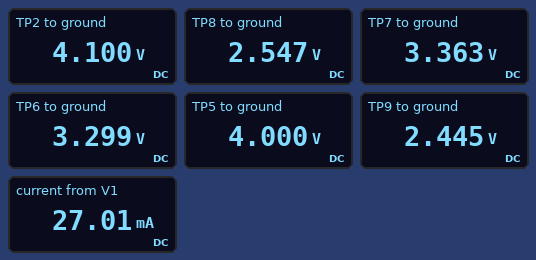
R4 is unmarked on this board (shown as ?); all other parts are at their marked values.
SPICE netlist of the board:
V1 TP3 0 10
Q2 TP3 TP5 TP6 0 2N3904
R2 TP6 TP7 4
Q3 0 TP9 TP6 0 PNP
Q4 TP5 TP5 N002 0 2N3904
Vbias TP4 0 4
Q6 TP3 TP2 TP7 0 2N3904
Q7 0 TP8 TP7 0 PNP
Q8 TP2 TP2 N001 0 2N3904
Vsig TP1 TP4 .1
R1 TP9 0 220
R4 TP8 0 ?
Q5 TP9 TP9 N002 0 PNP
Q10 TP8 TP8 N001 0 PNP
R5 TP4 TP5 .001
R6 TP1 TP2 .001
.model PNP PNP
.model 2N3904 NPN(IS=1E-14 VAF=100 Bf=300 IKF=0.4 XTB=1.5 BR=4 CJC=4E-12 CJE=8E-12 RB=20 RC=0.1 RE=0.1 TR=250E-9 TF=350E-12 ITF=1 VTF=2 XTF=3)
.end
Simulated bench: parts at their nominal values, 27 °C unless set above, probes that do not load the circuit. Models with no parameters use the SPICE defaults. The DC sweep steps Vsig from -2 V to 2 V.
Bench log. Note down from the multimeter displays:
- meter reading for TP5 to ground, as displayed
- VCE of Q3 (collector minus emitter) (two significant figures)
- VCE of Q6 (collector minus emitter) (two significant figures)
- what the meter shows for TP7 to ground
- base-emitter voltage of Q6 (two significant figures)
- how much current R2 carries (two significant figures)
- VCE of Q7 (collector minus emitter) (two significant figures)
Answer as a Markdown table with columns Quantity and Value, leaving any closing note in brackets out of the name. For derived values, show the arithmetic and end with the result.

| Quantity | Value |
|---|---|
| meter reading for TP5 to ground, as displayed | 4.000 V |
| VCE of Q3 (collector minus emitter) | 0 V - 3.299 V = -3.3 V |
| VCE of Q6 (collector minus emitter) | 10 V - 3.363 V = 6.6 V |
| what the meter shows for TP7 to ground | 3.363 V |
| base-emitter voltage of Q6 | 4.1 V - 3.363 V = 740 mV |
| how much current R2 carries | (3.363 V - 3.299 V) / 4 Ω = 16 mA |
| VCE of Q7 (collector minus emitter) | 0 V - 3.363 V = -3.4 V |
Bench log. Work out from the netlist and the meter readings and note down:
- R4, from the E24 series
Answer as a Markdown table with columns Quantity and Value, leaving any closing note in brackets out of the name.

| Quantity | Value |
|---|---|
| R4, from the E24 series | 240 Ω |
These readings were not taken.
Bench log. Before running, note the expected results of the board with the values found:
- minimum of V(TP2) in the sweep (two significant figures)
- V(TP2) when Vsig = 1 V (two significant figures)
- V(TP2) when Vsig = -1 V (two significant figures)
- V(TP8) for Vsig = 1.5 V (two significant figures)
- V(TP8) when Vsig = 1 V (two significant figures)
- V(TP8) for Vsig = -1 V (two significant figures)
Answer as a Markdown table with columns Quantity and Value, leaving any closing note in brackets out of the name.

| Quantity | Value |
|---|---|
| minimum of V(TP2) in the sweep | 2.0 V |
| V(TP2) when Vsig = 1 V | 5.0 V |
| V(TP2) when Vsig = -1 V | 3.0 V |
| V(TP8) for Vsig = 1.5 V | 3.9 V |
| V(TP8) when Vsig = 1 V | 3.4 V |
| V(TP8) for Vsig = -1 V | 1.5 V |
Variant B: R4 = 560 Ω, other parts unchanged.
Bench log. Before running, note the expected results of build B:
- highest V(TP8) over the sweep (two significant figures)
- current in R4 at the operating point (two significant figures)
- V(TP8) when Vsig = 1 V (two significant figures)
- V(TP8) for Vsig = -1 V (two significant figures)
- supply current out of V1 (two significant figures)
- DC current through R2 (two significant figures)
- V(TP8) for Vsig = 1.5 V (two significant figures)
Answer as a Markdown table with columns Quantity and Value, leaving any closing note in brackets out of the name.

| Quantity | Value |
|---|---|
| highest V(TP8) over the sweep | 4.5 V |
| current in R4 at the operating point | 4.6 mA |
| V(TP8) when Vsig = 1 V | 3.5 V |
| V(TP8) for Vsig = -1 V | 1.6 V |
| supply current out of V1 | 24 mA |
| DC current through R2 | 17 mA |
| V(TP8) for Vsig = 1.5 V | 4.0 V |
